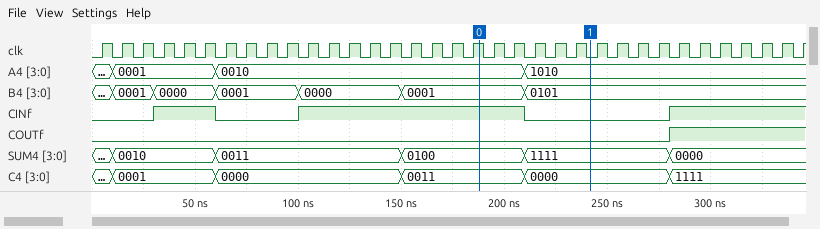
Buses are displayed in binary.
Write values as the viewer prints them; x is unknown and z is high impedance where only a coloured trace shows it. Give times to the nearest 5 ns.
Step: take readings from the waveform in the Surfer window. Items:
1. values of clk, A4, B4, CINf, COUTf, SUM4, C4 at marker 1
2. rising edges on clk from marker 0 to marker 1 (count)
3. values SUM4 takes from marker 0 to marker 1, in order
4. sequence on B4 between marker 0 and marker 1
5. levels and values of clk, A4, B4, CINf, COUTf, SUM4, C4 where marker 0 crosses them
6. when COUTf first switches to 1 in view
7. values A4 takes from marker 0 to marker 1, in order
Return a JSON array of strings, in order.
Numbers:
["clk=0, A4=1010, B4=0101, CINf=0, COUTf=0, SUM4=1111, C4=0000", "5", "0100, 1111", "0001, 0101", "clk=1, A4=0010, B4=0001, CINf=1, COUTf=0, SUM4=0100, C4=0011", "280 ns", "0010, 1010"]
